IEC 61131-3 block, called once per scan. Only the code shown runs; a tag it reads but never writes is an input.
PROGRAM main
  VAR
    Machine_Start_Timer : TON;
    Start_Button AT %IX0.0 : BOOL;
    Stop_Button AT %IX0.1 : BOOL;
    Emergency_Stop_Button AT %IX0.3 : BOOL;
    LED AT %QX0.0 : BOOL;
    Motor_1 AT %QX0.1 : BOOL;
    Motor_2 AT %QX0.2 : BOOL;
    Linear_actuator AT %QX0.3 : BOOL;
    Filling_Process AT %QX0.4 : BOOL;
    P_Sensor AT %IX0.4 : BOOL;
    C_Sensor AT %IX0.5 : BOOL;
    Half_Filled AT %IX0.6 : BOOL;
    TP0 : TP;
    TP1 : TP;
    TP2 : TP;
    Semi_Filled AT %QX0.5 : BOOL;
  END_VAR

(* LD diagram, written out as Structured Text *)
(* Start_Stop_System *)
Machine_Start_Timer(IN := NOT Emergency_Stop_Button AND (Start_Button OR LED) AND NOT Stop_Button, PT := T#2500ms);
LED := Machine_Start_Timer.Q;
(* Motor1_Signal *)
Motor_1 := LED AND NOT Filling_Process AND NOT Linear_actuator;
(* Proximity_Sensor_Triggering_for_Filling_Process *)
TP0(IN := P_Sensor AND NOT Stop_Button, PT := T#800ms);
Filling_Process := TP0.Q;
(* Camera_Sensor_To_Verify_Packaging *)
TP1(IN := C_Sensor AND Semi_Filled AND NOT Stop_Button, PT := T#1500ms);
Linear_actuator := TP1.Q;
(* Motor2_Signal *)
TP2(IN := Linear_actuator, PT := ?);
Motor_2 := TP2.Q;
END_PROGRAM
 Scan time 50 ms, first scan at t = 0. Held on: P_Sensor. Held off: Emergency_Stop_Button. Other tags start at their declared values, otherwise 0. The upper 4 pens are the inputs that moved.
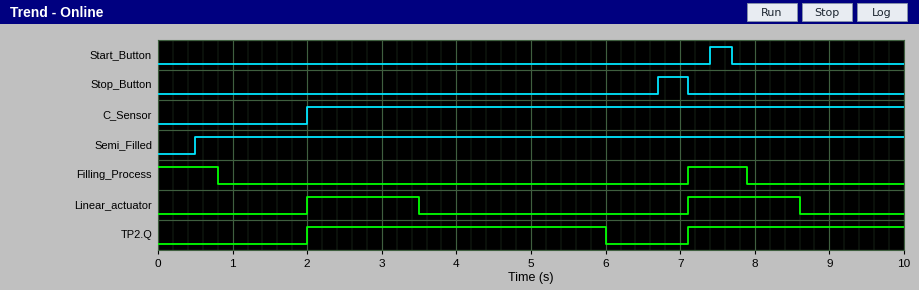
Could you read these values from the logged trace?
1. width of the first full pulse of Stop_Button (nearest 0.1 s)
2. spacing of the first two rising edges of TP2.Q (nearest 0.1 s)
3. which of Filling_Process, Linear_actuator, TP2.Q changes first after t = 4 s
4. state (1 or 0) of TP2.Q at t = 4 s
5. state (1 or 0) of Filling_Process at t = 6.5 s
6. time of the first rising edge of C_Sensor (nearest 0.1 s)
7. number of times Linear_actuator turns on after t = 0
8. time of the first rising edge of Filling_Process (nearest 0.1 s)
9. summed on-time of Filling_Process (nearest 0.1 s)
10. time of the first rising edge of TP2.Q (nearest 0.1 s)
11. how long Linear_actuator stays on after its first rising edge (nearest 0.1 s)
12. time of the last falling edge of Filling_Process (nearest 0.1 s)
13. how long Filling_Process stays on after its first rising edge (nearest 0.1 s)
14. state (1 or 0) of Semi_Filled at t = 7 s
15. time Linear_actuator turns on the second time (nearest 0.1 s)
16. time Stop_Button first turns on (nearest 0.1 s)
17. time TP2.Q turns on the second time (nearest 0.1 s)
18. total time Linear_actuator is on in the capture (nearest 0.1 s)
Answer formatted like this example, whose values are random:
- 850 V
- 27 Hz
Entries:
- 0.4 s
- 5.1 s
- TP2.Q
- 1
- 0
- 2.0 s
- 2
- 7.1 s
- 1.6 s
- 2.0 s
- 1.5 s
- 7.9 s
- 0.8 s
- 1
- 7.1 s
- 6.7 s
- 7.1 s
- 3.0 s
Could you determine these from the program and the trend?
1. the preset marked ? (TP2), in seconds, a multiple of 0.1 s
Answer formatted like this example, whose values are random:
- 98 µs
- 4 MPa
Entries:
- 4.0 s
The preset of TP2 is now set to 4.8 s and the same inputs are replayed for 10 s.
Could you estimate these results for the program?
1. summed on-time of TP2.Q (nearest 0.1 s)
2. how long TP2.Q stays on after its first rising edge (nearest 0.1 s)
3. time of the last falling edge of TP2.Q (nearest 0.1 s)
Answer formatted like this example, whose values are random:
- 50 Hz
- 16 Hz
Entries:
- 7.7 s
- 4.8 s
- 6.8 s
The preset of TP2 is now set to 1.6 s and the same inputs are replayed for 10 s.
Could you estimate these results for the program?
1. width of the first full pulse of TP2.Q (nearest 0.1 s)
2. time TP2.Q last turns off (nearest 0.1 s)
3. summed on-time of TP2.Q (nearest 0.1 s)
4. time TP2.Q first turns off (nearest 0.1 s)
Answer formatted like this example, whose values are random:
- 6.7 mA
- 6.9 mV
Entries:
- 1.6 s
- 8.7 s
- 3.2 s
- 3.6 s
